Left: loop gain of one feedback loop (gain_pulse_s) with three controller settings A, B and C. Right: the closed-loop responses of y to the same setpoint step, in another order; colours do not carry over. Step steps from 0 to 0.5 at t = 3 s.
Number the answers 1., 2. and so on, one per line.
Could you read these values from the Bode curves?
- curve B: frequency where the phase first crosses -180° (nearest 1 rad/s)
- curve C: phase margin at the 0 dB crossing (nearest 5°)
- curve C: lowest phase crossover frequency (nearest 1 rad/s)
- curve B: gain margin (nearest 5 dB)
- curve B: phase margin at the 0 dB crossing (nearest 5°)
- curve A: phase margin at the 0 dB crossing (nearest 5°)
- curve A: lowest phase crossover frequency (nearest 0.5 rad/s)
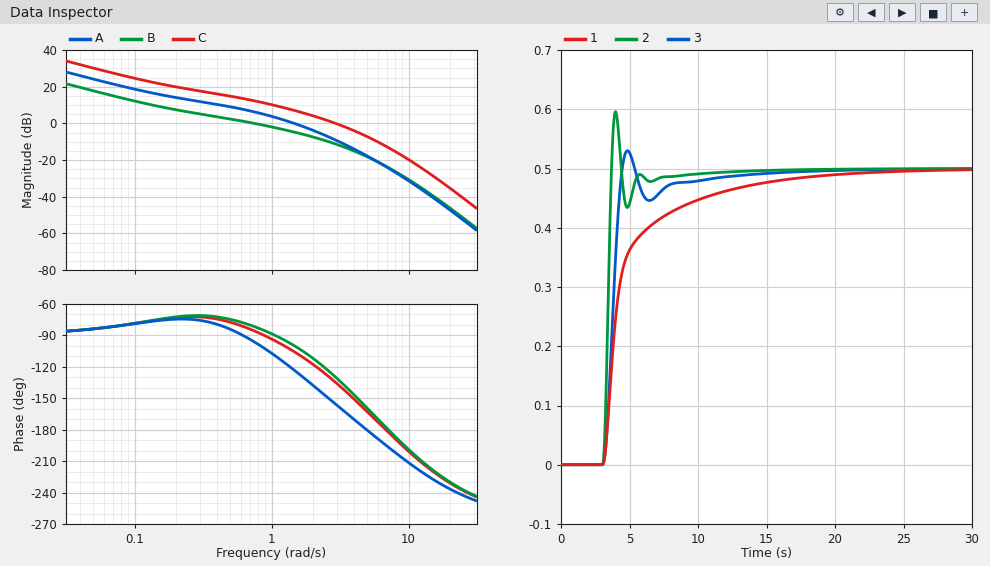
1. 7 rad/s
2. 45°
3. 7 rad/s
4. 25 dB
5. 100°
6. 55°
7. 5.0 rad/s
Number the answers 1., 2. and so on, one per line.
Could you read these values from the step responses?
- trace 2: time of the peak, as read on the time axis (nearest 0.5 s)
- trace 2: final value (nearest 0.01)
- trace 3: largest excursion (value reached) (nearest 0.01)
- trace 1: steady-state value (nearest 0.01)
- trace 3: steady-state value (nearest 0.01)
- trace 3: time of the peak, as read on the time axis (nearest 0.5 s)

1. 4.0 s
2. 0.50
3. 0.53
4. 0.50
5. 0.50
6. 5.0 s
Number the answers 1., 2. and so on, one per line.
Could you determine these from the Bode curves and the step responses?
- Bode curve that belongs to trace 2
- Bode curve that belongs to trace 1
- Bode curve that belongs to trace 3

1. C
2. B
3. A
